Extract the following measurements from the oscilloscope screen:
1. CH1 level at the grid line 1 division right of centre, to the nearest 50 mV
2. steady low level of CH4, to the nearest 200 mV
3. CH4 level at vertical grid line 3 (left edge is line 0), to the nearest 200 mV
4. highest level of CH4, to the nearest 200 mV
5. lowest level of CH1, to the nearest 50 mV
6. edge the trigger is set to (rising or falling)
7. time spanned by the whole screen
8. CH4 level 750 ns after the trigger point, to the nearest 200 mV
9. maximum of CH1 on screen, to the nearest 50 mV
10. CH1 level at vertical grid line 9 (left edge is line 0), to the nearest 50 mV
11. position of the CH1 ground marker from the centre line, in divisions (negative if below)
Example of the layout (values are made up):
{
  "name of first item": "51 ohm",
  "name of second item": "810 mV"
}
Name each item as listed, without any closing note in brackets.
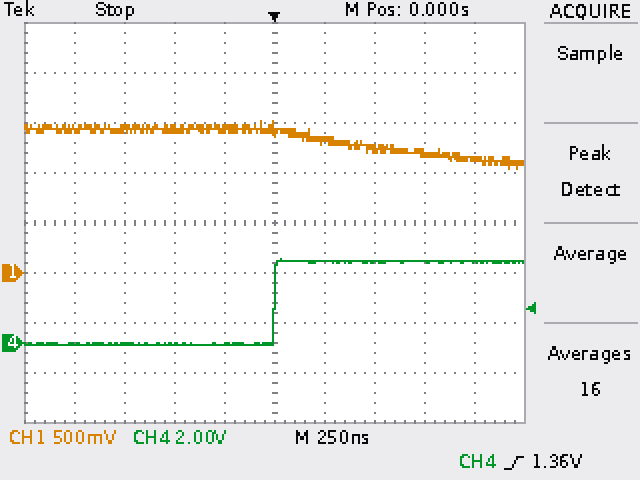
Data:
{
  "CH1 level at the grid line 1 division right of centre, to the nearest 50 mV": "1.30 V",
  "steady low level of CH4, to the nearest 200 mV": "0.0 V",
  "CH4 level at vertical grid line 3 (left edge is line 0), to the nearest 200 mV": "0.0 V",
  "highest level of CH4, to the nearest 200 mV": "3.4 V",
  "lowest level of CH1, to the nearest 50 mV": "1.05 V",
  "edge the trigger is set to": "rising",
  "time spanned by the whole screen": "2.5 µs",
  "CH4 level 750 ns after the trigger point, to the nearest 200 mV": "3.2 V",
  "maximum of CH1 on screen, to the nearest 50 mV": "1.50 V",
  "CH1 level at vertical grid line 9 (left edge is line 0), to the nearest 50 mV": "1.15 V",
  "position of the CH1 ground marker from the centre line, in divisions": "-1.0 div"
}
